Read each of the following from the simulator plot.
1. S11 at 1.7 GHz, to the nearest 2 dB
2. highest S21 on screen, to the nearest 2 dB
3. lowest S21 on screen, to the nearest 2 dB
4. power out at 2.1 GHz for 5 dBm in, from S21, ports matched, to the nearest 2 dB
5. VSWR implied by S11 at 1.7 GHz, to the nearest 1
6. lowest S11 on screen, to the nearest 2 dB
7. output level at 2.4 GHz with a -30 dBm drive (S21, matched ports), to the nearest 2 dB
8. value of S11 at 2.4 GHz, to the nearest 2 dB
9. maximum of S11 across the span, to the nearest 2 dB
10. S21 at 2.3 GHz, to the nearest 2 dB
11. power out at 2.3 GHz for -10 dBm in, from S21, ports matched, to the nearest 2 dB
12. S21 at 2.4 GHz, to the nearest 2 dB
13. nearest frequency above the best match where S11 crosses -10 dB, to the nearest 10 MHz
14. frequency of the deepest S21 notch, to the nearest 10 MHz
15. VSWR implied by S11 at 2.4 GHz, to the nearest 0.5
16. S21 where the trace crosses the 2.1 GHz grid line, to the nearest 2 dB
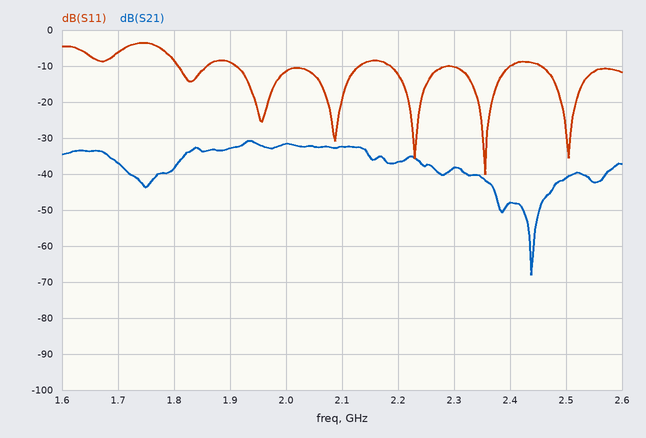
-6 dB
-30 dB
-68 dB
-28 dBm
3
-40 dB
-78 dBm
-10 dB
-4 dB
-38 dB
-48 dBm
-48 dB
2.40 GHz
2.44 GHz
2.0
-32 dB
